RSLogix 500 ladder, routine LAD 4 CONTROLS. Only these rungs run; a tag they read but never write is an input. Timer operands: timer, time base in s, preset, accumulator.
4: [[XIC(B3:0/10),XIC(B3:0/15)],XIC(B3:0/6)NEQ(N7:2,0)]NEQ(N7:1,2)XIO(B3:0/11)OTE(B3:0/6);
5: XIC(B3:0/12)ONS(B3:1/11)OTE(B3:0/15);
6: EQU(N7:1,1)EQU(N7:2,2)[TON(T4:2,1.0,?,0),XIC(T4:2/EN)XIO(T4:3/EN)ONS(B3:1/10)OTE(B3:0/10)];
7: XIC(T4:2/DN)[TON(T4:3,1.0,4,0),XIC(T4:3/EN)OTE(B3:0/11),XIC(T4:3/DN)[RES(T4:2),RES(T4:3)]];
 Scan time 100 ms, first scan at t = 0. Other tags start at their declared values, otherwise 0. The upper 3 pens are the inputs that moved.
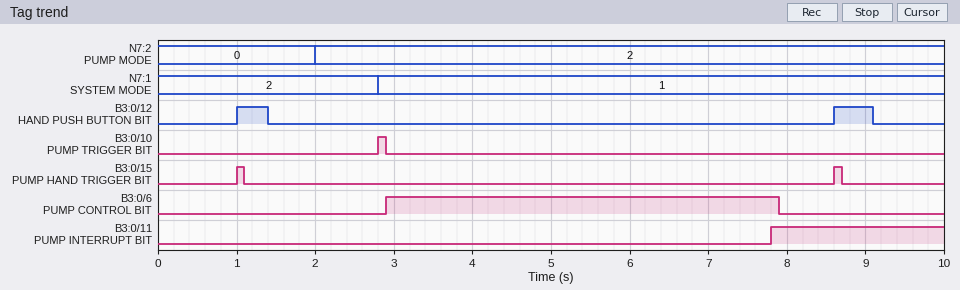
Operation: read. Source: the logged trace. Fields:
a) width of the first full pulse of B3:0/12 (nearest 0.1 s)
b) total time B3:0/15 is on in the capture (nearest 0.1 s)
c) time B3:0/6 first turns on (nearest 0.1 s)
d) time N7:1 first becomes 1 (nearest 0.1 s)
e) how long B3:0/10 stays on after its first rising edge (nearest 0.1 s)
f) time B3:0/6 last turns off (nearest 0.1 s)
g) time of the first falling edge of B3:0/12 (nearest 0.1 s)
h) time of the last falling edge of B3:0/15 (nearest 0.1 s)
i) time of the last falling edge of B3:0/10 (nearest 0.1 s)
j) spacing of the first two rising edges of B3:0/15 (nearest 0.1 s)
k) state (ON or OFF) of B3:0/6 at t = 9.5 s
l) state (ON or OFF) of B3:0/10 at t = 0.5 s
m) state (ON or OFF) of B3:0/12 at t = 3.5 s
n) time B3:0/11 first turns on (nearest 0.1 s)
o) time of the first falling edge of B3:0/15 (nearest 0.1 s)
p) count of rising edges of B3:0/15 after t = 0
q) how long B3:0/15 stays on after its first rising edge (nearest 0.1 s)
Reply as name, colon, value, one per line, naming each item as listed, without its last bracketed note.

width of the first full pulse of B3:0/12: 0.4 s
total time B3:0/15 is on in the capture: 0.2 s
time B3:0/6 first turns on: 2.9 s
time N7:1 first becomes 1: 2.8 s
how long B3:0/10 stays on after its first rising edge: 0.1 s
time B3:0/6 last turns off: 7.9 s
time of the first falling edge of B3:0/12: 1.4 s
time of the last falling edge of B3:0/15: 8.7 s
time of the last falling edge of B3:0/10: 2.9 s
spacing of the first two rising edges of B3:0/15: 7.6 s
state (ON or OFF) of B3:0/6 at t = 9.5 s: OFF
state (ON or OFF) of B3:0/10 at t = 0.5 s: OFF
state (ON or OFF) of B3:0/12 at t = 3.5 s: OFF
time B3:0/11 first turns on: 7.8 s
time of the first falling edge of B3:0/15: 1.1 s
count of rising edges of B3:0/15 after t = 0: 2
how long B3:0/15 stays on after its first rising edge: 0.1 s
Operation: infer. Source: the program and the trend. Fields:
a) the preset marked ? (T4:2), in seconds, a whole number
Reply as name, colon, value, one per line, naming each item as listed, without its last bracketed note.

the preset marked ? (T4:2), in seconds, a whole number: 5 s
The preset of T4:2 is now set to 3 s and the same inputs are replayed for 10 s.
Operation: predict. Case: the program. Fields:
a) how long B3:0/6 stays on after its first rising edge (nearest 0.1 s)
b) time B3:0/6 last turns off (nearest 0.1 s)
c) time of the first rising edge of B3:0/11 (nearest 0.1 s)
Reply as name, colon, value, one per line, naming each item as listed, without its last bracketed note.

how long B3:0/6 stays on after its first rising edge: 3.0 s
time B3:0/6 last turns off: 5.9 s
time of the first rising edge of B3:0/11: 5.8 s
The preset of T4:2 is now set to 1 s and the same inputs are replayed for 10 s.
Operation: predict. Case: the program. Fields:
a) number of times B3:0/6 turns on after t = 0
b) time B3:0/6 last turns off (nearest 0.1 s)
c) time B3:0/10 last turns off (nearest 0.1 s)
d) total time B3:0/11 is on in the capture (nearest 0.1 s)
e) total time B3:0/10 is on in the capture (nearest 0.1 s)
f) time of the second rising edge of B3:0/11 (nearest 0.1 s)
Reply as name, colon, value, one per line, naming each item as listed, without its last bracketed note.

number of times B3:0/6 turns on after t = 0: 2
time B3:0/6 last turns off: 9.0 s
time B3:0/10 last turns off: 8.0 s
total time B3:0/11 is on in the capture: 5.2 s
total time B3:0/10 is on in the capture: 0.2 s
time of the second rising edge of B3:0/11: 8.9 s
